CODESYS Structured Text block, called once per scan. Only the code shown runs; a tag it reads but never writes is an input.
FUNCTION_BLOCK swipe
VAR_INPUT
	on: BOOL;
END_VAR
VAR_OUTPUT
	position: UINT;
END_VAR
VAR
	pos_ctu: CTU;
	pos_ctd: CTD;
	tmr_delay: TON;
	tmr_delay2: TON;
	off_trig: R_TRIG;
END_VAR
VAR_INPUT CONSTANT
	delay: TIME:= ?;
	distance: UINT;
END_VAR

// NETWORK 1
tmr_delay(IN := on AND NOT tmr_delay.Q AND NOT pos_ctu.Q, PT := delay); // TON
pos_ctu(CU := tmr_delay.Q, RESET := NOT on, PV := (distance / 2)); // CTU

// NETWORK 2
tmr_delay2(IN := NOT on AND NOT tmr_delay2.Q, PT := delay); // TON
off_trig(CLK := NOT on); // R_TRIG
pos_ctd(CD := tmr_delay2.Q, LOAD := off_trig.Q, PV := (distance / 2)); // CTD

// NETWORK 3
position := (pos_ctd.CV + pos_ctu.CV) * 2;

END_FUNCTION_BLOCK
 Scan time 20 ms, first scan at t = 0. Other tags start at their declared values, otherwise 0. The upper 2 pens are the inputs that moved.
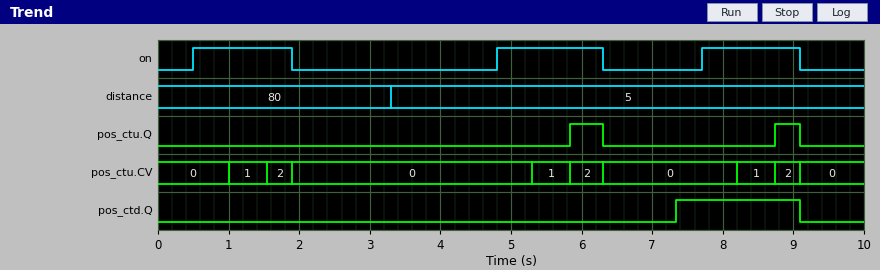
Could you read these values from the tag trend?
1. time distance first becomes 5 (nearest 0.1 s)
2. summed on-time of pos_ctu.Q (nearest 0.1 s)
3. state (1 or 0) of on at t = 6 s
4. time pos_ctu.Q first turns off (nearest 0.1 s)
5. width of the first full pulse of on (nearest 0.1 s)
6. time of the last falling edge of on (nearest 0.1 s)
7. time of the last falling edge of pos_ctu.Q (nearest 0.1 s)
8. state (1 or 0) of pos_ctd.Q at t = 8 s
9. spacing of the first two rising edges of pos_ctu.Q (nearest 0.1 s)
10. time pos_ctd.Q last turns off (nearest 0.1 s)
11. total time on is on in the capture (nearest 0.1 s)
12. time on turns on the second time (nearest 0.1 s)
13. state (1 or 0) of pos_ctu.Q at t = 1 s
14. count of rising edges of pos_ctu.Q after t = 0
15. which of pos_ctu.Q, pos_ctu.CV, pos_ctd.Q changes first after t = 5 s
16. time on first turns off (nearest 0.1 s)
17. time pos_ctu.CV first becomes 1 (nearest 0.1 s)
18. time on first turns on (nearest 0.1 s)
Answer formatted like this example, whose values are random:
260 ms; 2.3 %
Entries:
3.3 s; 0.8 s; 1; 6.3 s; 1.4 s; 9.1 s; 9.1 s; 1; 2.9 s; 9.1 s; 4.3 s; 4.8 s; 0; 2; pos_ctu.CV; 1.9 s; 1.0 s; 0.5 s
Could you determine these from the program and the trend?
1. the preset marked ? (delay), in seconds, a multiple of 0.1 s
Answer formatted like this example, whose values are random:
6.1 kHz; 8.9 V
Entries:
0.5 s
